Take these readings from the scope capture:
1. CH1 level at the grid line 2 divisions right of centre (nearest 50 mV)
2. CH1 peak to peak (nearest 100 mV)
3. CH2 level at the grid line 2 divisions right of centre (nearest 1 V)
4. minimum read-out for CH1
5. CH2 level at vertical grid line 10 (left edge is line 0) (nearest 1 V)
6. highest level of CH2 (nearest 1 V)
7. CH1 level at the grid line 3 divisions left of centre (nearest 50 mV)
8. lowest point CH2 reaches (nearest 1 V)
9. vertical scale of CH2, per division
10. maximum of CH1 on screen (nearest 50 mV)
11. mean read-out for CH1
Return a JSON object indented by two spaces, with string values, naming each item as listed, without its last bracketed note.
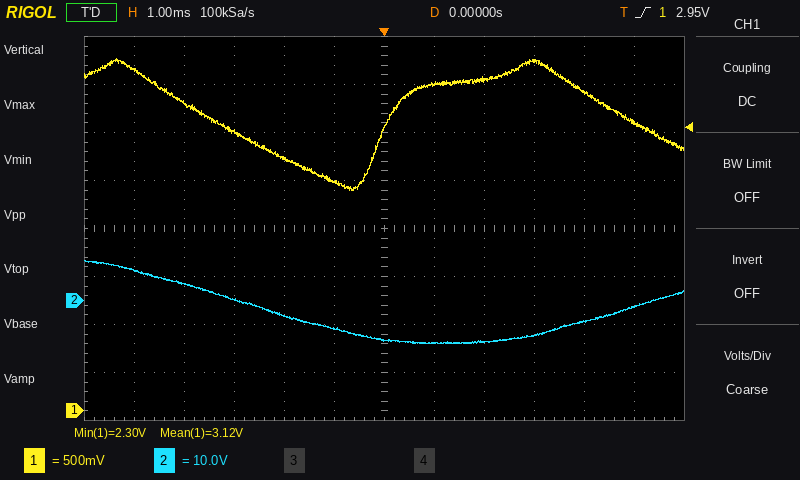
{
  "CH1 level at the grid line 2 divisions right of centre": "3.45 V",
  "CH1 peak to peak": "1.40 V",
  "CH2 level at the grid line 2 divisions right of centre": "-9 V",
  "minimum read-out for CH1": "2.30 V",
  "CH2 level at vertical grid line 10 (left edge is line 0)": "-4 V",
  "highest level of CH2": "8 V",
  "CH1 level at the grid line 3 divisions left of centre": "2.90 V",
  "lowest point CH2 reaches": "-9 V",
  "vertical scale of CH2, per division": "10 V",
  "maximum of CH1 on screen": "3.65 V",
  "mean read-out for CH1": "3.12 V"
}
